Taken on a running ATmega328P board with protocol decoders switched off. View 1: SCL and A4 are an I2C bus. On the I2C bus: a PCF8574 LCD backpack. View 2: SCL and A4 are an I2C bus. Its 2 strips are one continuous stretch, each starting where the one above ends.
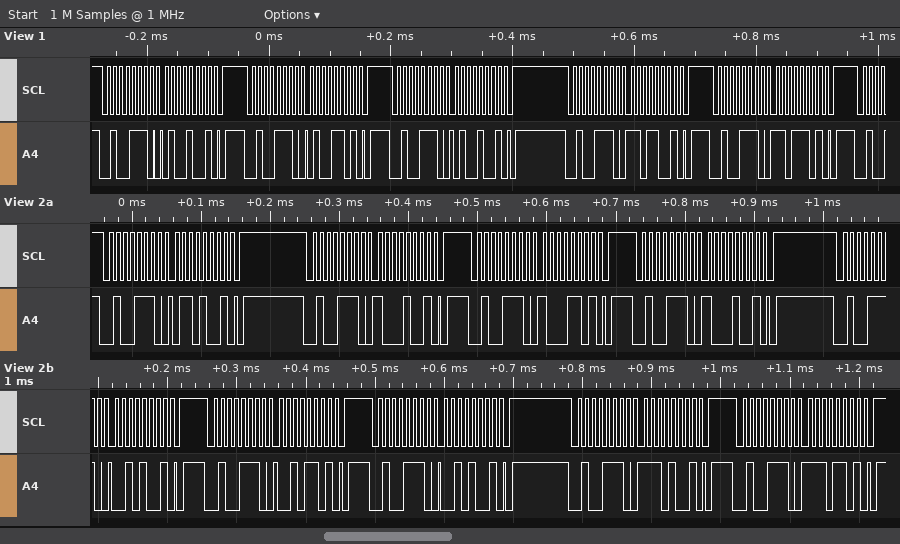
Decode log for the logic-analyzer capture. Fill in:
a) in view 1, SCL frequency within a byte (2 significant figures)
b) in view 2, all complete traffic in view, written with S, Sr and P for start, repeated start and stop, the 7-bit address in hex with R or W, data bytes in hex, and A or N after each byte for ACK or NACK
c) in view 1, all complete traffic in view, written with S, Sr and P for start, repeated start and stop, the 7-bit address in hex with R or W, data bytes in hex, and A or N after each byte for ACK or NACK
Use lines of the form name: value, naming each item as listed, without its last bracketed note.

in view 1, SCL frequency within a byte: 100 kHz
in view 2, all complete traffic in view, written with S, Sr and P for start, repeated start and stop, the 7-bit address in hex with R or W, data bytes in hex, and A or N after each byte for ACK or NACK: S 27W A 69 A P S 27W A 89 A P S 27W A 8D A P S 27W A 89 A P S 27W A 29 A P S 27W A 2D A P S 27W A 29 A P S 27W A E9 A P S 27W A ED A P
in view 1, all complete traffic in view, written with S, Sr and P for start, repeated start and stop, the 7-bit address in hex with R or W, data bytes in hex, and A or N after each byte for ACK or NACK: S 27W A 49 A P S 27W A 4D A P S 27W A 49 A P S 27W A D9 A P S 27W A DD A P
